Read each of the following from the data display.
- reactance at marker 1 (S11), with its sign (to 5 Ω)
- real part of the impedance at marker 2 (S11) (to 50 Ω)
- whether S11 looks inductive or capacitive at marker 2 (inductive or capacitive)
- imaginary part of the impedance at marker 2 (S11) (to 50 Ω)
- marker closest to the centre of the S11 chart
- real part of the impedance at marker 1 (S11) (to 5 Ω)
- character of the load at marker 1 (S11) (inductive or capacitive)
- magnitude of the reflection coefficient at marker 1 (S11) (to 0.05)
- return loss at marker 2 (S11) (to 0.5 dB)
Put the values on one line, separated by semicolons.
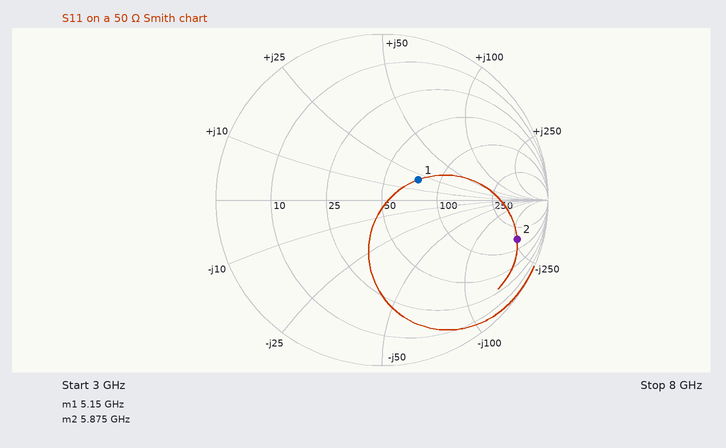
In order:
+20 Ω; 150 Ω; capacitive; -250 Ω; marker 1; 75 Ω; inductive; 0.25; 1.5 dB
